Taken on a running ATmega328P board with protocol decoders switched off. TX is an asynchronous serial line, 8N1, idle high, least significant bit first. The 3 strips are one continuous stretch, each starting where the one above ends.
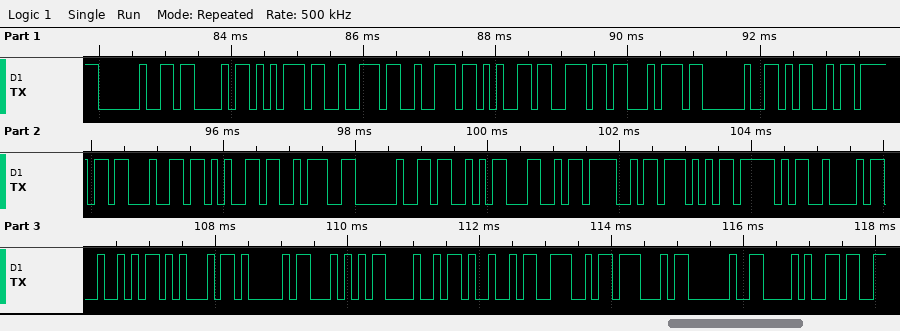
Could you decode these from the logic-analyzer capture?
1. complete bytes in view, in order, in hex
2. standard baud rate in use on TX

0x20 0x43 0x75 0x72 0x72 0x65 0x6E 0x74 0x20 0x4D 0x6F 0x64 0x65 0x3A 0x20 0x53 0x4C 0x4F 0x57 0x5F 0x42 0x52 0x45 0x41 0x54 0x48 0x49 0x4E 0x47 0x20 0x28
9600 baud
